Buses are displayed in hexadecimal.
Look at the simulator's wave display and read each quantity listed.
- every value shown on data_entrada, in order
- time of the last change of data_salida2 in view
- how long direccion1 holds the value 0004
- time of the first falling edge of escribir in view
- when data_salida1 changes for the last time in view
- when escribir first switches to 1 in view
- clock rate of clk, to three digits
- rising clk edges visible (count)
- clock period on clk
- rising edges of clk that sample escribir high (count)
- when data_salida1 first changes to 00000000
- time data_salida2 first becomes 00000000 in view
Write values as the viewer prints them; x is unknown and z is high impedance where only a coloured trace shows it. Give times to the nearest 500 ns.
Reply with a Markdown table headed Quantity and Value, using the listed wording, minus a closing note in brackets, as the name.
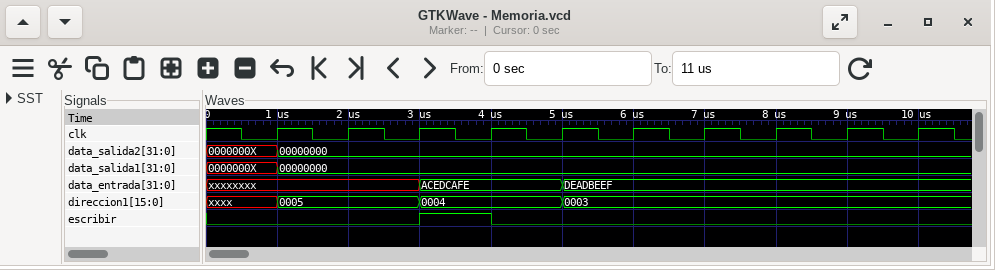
| Quantity | Value |
|---|---|
| every value shown on data_entrada, in order | xxxxxxxx, ACEDCAFE, DEADBEEF |
| time of the last change of data_salida2 in view | 1000 ns |
| how long direccion1 holds the value 0004 | 2000 ns |
| time of the first falling edge of escribir in view | 4000 ns |
| when data_salida1 changes for the last time in view | 1000 ns |
| when escribir first switches to 1 in view | 3000 ns |
| clock rate of clk, to three digits | 1.00 MHz |
| rising clk edges visible | 10 |
| clock period on clk | 1000 ns |
| rising edges of clk that sample escribir high | 1 |
| when data_salida1 first changes to 00000000 | 1000 ns |
| time data_salida2 first becomes 00000000 in view | 1000 ns |
